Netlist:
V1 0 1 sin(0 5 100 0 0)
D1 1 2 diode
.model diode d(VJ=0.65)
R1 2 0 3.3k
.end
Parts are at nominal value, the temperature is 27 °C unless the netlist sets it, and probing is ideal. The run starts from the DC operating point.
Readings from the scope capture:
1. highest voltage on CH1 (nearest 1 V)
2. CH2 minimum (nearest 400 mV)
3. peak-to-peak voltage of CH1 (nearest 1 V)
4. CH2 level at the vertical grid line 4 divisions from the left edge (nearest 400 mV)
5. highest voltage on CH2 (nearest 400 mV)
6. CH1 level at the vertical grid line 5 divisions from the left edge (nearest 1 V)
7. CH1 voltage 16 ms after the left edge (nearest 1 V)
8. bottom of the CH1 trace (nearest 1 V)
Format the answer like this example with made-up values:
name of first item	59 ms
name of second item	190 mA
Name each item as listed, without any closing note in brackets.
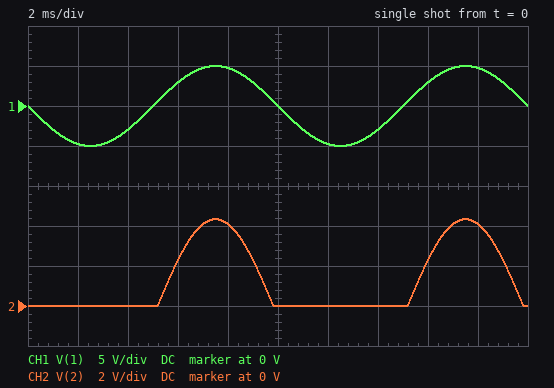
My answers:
highest voltage on CH1	5 V
CH2 minimum	0 V
peak-to-peak voltage of CH1	10 V
CH2 level at the vertical grid line 4 divisions from the left edge	4.0 V
highest voltage on CH2	4.4 V
CH1 level at the vertical grid line 5 divisions from the left edge	0 V
CH1 voltage 16 ms after the left edge	3 V
bottom of the CH1 trace	-5 V
